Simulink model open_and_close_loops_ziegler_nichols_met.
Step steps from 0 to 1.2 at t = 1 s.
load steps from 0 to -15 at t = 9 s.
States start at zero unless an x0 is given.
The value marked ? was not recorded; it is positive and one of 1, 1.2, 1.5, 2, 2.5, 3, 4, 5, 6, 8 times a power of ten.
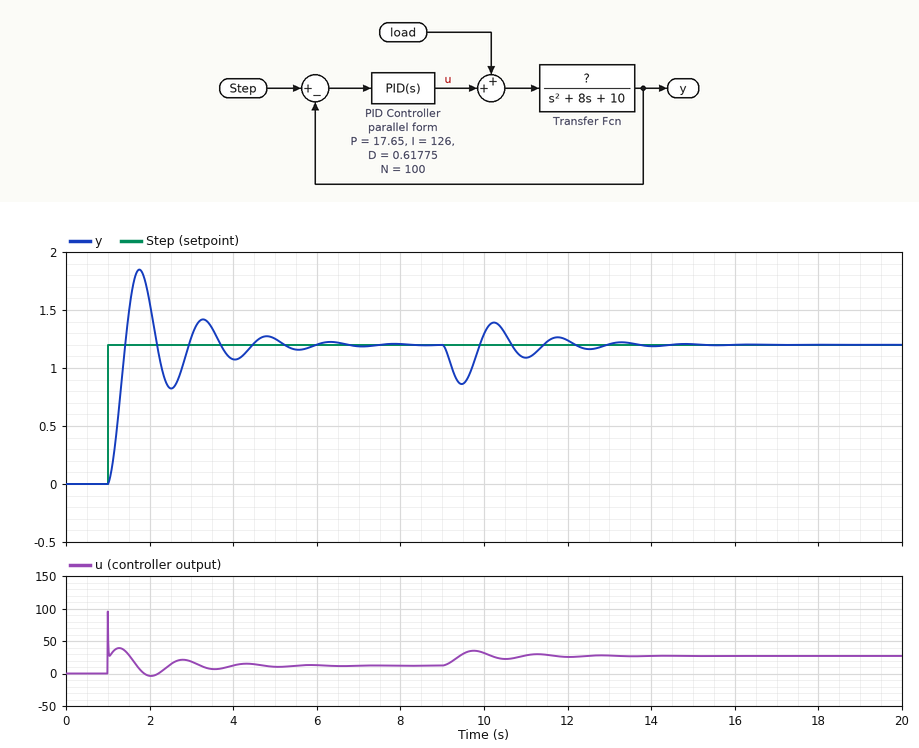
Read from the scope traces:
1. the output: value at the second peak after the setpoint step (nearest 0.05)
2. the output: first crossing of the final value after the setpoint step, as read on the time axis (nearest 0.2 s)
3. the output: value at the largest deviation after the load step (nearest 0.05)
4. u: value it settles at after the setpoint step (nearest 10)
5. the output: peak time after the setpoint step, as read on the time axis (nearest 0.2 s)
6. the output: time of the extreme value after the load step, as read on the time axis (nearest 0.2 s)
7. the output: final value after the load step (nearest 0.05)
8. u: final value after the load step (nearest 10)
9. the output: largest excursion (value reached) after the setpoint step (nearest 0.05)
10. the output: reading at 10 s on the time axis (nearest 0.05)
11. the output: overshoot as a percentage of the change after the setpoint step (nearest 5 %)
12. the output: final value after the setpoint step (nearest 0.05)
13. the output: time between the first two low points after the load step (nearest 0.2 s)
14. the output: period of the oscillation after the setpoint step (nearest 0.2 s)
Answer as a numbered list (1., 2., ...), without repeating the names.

1. 1.40
2. 1.4 s
3. 0.85
4. 10
5. 1.8 s
6. 9.4 s
7. 1.20
8. 30
9. 1.85
10. 1.30
11. 55 %
12. 1.20
13. 1.6 s
14. 1.6 s
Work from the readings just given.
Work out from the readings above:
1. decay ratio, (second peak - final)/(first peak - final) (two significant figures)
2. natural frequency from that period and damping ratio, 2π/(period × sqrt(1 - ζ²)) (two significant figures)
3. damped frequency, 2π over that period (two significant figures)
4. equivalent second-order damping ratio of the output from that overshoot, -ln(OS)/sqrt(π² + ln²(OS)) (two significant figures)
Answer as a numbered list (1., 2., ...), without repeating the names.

1. 0.31
2. 4.0 rad/s
3. 3.9 rad/s
4. 0.19
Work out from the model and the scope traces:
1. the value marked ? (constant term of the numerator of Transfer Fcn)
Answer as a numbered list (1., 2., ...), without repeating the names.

1. 1
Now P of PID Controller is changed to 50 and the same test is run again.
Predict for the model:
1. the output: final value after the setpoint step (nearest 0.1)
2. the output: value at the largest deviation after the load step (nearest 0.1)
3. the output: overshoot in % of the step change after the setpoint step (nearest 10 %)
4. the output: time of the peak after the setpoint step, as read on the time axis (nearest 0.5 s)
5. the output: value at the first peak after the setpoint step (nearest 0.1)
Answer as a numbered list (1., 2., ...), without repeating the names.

1. 1.2
2. 1.0
3. 30 %
4. 1.5 s
5. 1.5
